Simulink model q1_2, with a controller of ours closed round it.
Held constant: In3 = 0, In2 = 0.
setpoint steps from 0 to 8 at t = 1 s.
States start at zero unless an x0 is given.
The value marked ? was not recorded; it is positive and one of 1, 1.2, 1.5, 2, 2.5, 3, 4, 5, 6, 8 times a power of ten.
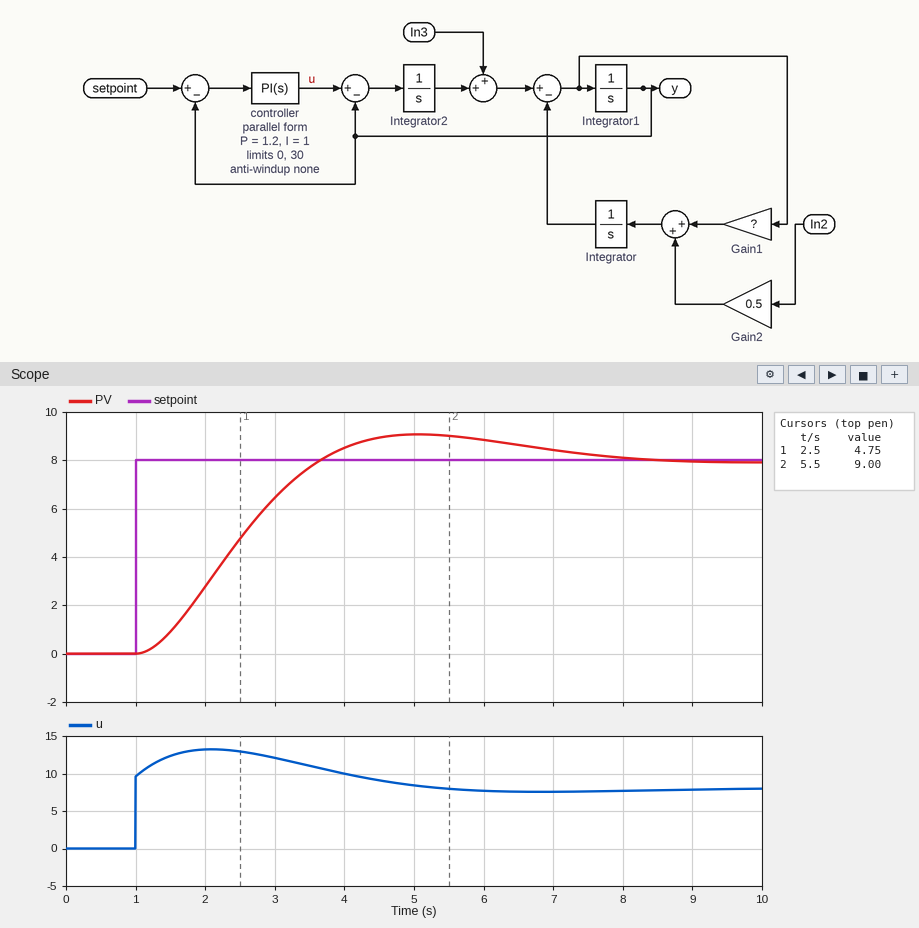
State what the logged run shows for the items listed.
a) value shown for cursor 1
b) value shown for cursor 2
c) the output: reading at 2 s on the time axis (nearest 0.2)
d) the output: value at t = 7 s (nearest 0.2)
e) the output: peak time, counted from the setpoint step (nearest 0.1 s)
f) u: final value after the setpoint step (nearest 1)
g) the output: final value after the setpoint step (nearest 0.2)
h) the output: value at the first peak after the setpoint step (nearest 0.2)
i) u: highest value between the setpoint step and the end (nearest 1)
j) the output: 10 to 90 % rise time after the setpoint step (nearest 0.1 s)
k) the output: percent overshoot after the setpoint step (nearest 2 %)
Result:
4.75
9.00
2.8
8.4
4.1 s
8
8.0
9.0
13
1.8 s
14 %
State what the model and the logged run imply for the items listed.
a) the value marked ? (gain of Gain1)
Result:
2.5
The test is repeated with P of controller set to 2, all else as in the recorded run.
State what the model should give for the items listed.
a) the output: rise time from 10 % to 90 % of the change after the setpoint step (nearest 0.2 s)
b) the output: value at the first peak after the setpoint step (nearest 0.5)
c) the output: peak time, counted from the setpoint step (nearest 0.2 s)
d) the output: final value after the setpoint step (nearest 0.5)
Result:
1.6 s
8.5
3.2 s
8.0
